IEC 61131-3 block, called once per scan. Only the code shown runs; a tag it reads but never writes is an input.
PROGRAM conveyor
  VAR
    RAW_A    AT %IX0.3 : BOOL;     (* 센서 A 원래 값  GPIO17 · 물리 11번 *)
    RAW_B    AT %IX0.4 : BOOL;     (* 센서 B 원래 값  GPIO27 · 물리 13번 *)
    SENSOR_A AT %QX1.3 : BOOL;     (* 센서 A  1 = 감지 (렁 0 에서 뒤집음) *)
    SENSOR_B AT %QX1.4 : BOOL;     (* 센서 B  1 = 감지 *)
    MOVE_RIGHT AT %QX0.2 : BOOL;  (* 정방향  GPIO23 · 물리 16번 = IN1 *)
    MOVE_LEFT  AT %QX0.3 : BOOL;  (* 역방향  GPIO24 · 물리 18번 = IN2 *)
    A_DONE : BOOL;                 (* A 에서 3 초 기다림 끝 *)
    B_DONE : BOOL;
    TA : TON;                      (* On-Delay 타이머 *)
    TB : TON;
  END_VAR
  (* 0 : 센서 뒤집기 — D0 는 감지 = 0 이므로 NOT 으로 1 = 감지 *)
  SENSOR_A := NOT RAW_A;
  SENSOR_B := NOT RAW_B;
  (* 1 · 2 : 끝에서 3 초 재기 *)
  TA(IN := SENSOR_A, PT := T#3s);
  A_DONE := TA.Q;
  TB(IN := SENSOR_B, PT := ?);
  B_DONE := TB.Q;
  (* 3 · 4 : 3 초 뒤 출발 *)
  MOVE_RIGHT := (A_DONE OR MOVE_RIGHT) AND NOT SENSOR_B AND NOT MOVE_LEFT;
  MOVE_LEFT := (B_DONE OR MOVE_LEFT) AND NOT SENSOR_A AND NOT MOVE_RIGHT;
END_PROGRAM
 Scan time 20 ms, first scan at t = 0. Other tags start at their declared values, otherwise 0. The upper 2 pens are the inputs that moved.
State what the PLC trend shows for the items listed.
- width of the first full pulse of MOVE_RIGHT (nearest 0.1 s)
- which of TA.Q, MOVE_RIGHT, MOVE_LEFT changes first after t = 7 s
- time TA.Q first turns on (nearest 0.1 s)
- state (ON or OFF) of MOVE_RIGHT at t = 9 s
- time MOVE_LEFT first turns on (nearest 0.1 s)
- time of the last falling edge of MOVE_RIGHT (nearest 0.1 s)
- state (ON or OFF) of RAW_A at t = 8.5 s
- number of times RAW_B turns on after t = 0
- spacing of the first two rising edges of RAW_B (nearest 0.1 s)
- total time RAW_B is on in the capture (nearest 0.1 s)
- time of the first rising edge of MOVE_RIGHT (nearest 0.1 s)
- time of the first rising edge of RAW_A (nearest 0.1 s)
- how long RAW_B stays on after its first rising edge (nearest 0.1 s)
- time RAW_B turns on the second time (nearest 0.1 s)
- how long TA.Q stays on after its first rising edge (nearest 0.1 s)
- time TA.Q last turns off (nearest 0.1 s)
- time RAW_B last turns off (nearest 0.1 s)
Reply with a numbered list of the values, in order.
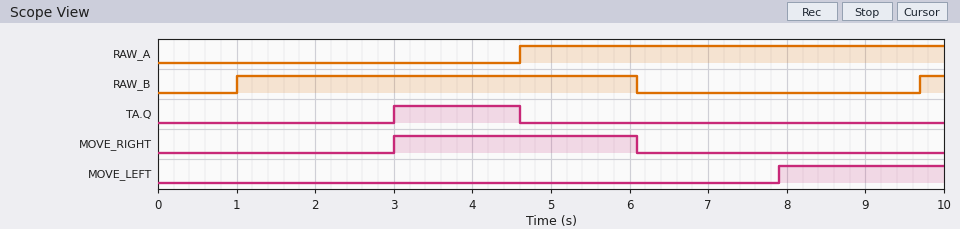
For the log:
1. 3.1 s
2. MOVE_LEFT
3. 3.0 s
4. OFF
5. 7.9 s
6. 6.1 s
7. ON
8. 2
9. 8.7 s
10. 5.4 s
11. 3.0 s
12. 4.6 s
13. 5.1 s
14. 9.7 s
15. 1.6 s
16. 4.6 s
17. 6.1 s
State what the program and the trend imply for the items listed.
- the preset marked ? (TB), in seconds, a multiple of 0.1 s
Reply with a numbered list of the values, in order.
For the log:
1. 1.8 s
